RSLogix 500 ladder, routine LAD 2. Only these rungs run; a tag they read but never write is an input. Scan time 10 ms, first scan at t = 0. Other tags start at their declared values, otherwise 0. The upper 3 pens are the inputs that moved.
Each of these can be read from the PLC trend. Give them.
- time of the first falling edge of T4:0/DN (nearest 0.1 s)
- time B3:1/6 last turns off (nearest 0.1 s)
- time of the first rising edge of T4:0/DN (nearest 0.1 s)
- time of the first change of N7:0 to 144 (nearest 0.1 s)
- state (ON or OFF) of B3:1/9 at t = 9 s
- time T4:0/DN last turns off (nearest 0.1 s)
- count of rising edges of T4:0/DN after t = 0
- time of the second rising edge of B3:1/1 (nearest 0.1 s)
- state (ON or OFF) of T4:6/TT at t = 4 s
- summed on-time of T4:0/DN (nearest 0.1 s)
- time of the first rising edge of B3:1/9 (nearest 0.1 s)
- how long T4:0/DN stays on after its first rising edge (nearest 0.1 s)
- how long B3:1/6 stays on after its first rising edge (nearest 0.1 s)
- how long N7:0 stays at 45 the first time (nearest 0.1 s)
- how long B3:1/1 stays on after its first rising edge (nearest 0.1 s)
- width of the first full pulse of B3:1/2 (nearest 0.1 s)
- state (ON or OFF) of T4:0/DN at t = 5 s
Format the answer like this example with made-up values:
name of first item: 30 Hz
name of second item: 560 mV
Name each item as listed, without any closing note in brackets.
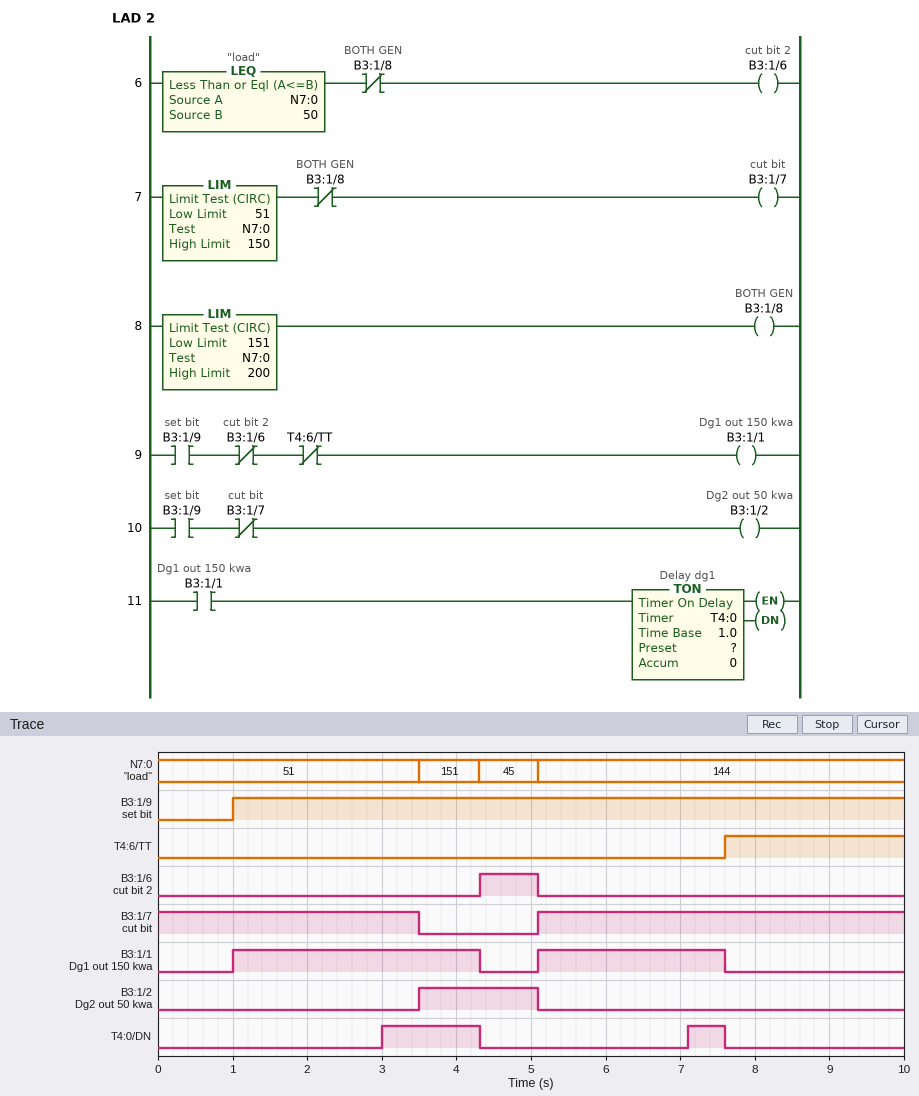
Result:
time of the first falling edge of T4:0/DN: 4.3 s
time B3:1/6 last turns off: 5.1 s
time of the first rising edge of T4:0/DN: 3.0 s
time of the first change of N7:0 to 144: 5.1 s
state (ON or OFF) of B3:1/9 at t = 9 s: ON
time T4:0/DN last turns off: 7.6 s
count of rising edges of T4:0/DN after t = 0: 2
time of the second rising edge of B3:1/1: 5.1 s
state (ON or OFF) of T4:6/TT at t = 4 s: OFF
summed on-time of T4:0/DN: 1.8 s
time of the first rising edge of B3:1/9: 1.0 s
how long T4:0/DN stays on after its first rising edge: 1.3 s
how long B3:1/6 stays on after its first rising edge: 0.8 s
how long N7:0 stays at 45 the first time: 0.8 s
how long B3:1/1 stays on after its first rising edge: 3.3 s
width of the first full pulse of B3:1/2: 1.6 s
state (ON or OFF) of T4:0/DN at t = 5 s: OFF
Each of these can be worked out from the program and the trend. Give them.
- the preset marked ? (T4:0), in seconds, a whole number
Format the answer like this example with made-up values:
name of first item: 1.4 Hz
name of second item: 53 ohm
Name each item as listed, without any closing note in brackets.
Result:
the preset marked ? (T4:0), in seconds, a whole number: 2 s
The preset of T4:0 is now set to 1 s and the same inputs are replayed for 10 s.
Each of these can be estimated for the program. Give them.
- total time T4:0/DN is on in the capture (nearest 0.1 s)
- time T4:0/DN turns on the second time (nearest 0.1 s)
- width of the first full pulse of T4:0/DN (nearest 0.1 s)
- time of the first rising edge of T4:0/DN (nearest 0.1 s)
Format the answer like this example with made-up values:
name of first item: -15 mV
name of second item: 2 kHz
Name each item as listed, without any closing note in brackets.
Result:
total time T4:0/DN is on in the capture: 3.8 s
time T4:0/DN turns on the second time: 6.1 s
width of the first full pulse of T4:0/DN: 2.3 s
time of the first rising edge of T4:0/DN: 2.0 s
